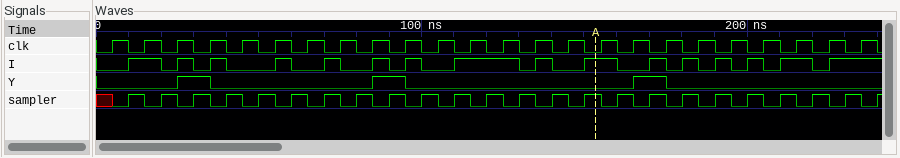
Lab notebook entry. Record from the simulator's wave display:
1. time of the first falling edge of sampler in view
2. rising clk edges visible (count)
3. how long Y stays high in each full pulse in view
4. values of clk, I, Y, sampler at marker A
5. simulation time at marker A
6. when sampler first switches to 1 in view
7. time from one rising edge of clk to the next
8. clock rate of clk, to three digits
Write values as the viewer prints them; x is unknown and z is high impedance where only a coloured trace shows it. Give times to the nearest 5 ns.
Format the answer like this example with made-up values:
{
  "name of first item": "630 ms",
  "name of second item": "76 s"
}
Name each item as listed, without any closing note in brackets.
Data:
{
  "time of the first falling edge of sampler in view": "15 ns",
  "rising clk edges visible": "24",
  "how long Y stays high in each full pulse in view": "10 ns, 10 ns, 10 ns",
  "values of clk, I, Y, sampler at marker A": "clk=0, I=1, Y=0, sampler=1",
  "simulation time at marker A": "155 ns",
  "when sampler first switches to 1 in view": "10 ns",
  "time from one rising edge of clk to the next": "10 ns",
  "clock rate of clk, to three digits": "100 MHz"
}
